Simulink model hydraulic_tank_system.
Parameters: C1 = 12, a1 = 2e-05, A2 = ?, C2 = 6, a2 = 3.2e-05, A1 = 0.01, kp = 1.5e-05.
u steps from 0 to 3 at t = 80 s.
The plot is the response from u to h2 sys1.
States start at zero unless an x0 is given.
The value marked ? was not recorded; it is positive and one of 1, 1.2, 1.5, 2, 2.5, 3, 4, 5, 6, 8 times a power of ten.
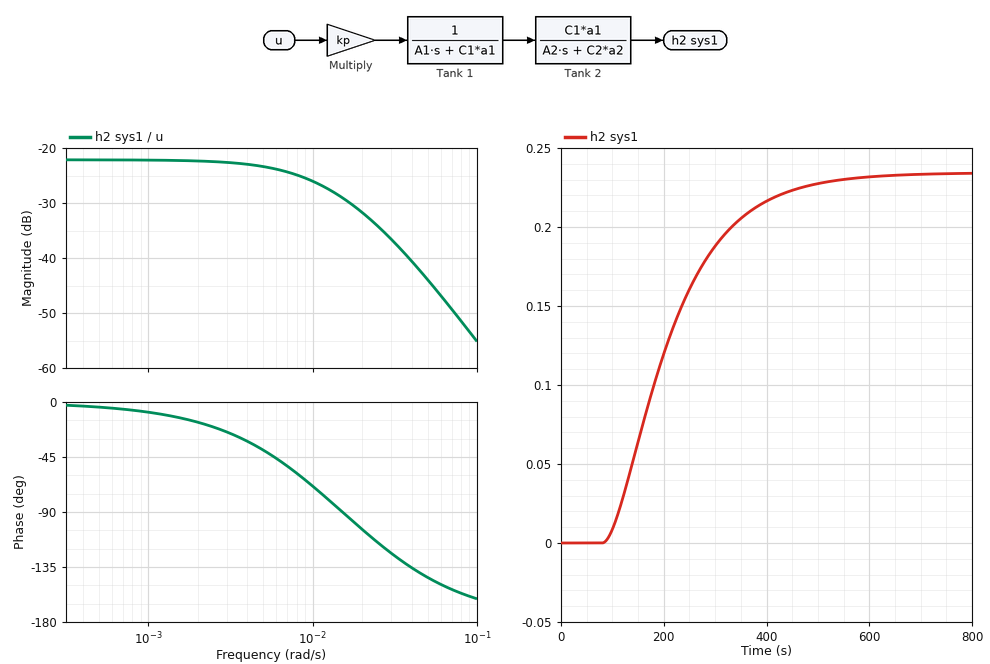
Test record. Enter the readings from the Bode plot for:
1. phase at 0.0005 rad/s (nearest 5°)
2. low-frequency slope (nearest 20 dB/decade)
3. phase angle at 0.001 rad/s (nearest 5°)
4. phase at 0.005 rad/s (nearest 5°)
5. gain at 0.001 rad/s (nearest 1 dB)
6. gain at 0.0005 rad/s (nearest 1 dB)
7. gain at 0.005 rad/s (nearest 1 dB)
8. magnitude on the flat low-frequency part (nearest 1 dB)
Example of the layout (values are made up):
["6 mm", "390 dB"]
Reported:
["-5°", "0 dB/decade", "-10°", "-40°", "-22 dB", "-22 dB", "-23 dB", "-22 dB"]
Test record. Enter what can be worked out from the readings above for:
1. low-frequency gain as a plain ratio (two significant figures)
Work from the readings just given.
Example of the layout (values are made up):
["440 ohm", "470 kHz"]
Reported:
["0.079"]
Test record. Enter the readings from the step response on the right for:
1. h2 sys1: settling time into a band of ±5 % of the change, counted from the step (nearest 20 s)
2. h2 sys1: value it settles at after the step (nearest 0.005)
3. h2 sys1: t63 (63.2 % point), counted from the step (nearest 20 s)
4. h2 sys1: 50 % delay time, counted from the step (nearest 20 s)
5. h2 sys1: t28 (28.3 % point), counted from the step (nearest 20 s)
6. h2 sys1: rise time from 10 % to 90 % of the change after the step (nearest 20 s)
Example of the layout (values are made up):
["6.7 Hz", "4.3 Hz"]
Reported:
["360 s", "0.235", "160 s", "120 s", "80 s", "260 s"]
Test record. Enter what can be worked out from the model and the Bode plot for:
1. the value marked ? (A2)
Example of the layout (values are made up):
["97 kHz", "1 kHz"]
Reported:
["0.02"]
